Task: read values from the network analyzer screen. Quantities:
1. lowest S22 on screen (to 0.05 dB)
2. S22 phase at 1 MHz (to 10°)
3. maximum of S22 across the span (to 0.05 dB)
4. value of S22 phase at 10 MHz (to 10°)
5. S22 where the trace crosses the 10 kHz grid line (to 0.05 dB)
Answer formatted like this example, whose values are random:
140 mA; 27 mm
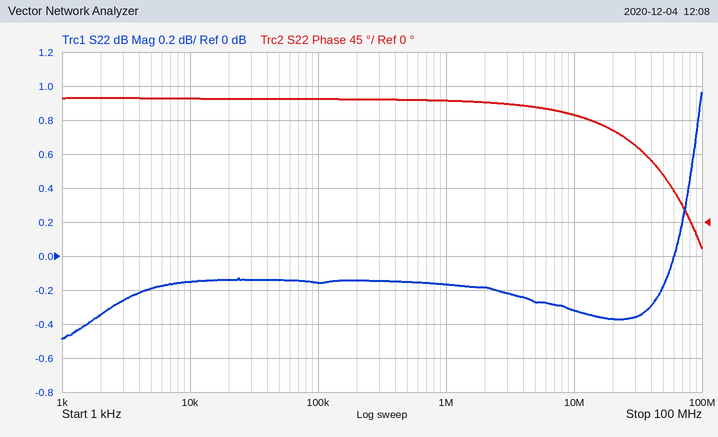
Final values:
-0.50 dB; 160°; 0.95 dB; 140°; -0.15 dB
